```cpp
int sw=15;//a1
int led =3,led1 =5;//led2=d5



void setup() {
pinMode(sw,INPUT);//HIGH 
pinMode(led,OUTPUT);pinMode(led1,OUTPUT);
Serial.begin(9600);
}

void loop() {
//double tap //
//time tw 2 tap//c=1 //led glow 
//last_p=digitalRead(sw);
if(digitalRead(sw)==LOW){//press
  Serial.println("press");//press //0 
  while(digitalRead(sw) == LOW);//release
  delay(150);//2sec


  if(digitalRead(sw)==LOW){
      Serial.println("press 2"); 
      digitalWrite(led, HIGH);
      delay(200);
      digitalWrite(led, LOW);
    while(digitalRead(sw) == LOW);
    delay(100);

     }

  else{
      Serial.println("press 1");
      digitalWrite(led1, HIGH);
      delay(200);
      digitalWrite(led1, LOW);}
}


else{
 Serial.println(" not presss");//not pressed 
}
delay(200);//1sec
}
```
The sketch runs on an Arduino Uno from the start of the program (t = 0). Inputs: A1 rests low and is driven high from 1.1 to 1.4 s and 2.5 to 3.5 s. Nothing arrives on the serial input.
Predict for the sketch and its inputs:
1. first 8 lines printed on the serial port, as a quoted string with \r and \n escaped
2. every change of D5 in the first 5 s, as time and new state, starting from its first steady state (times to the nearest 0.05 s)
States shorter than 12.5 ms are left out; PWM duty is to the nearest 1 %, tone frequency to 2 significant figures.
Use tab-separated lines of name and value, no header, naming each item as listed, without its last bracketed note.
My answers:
first 8 lines printed on the serial port, as a quoted string with \r and \n escaped	"press\r\npress 1\r\npress\r\npress 1\r\n not presss\r\n not presss\r\n not presss\r\npress\r\n"
every change of D5 in the first 5 s, as time and new state, starting from its first steady state	0 s low; 1.25 s high; 1.45 s low; 2.65 s high; 2.85 s low
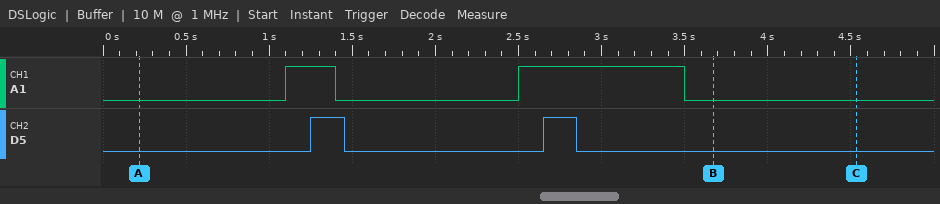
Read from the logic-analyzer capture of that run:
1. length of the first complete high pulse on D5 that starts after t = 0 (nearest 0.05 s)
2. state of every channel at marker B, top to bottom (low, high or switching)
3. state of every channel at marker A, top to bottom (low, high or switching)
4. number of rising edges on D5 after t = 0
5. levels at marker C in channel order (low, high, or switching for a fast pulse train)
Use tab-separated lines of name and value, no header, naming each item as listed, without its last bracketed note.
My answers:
length of the first complete high pulse on D5 that starts after t = 0	0.20 s
state of every channel at marker B, top to bottom	A1 low, D5 low
state of every channel at marker A, top to bottom	A1 low, D5 low
number of rising edges on D5 after t = 0	2
levels at marker C in channel order	A1 low, D5 low
